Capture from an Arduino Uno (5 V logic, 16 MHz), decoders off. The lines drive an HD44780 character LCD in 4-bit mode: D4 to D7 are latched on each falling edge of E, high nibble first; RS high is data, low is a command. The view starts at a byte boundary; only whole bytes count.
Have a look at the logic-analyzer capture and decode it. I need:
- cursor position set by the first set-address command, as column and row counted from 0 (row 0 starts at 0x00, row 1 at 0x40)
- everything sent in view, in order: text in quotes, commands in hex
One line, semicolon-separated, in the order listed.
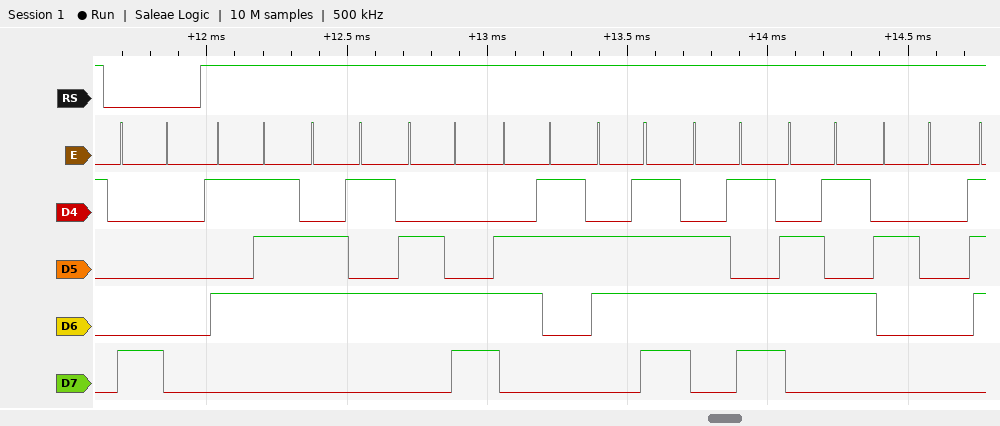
column 0, row 0; 0x80 "Welcome "
